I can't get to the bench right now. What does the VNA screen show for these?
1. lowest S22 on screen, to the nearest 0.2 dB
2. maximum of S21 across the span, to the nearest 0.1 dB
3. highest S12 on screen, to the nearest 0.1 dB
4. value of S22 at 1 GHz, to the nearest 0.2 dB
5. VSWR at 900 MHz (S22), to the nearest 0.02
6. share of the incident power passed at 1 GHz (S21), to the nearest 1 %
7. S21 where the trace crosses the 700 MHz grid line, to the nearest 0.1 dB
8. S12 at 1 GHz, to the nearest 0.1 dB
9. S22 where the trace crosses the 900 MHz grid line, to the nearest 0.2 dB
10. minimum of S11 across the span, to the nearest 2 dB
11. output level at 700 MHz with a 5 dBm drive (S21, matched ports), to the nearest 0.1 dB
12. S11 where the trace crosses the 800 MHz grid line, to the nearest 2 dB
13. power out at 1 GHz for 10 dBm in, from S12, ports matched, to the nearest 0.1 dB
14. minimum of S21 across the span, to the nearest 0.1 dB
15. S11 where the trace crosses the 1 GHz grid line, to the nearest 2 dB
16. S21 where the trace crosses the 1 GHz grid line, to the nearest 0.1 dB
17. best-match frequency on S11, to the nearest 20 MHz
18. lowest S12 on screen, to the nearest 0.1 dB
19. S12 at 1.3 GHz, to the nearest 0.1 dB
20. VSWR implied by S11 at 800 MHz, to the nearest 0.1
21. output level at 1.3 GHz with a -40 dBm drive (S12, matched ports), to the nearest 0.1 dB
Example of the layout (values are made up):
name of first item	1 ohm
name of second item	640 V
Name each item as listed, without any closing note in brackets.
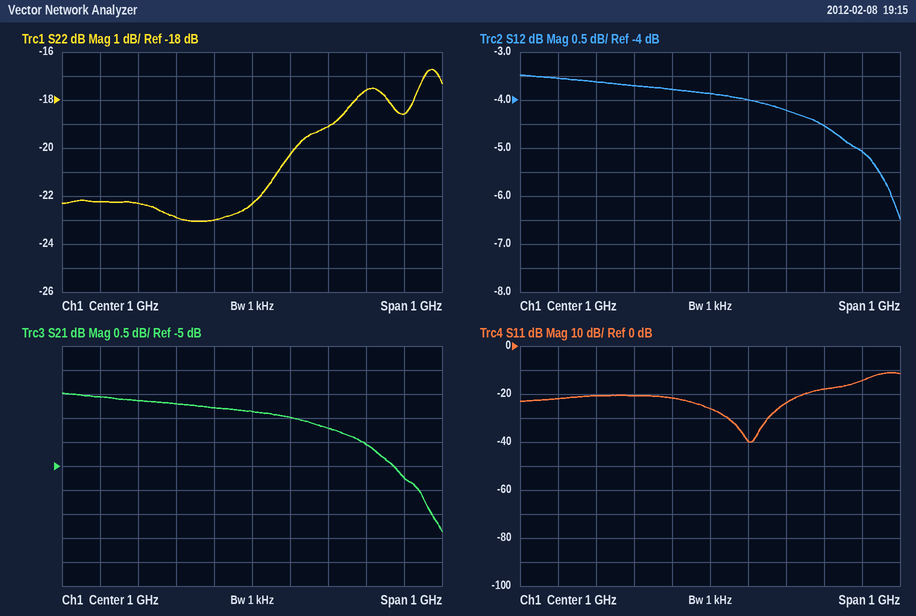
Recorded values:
lowest S22 on screen, to the nearest 0.2 dB	-23.0 dB
maximum of S21 across the span, to the nearest 0.1 dB	-3.5 dB
highest S12 on screen, to the nearest 0.1 dB	-3.5 dB
value of S22 at 1 GHz, to the nearest 0.2 dB	-22.4 dB
VSWR at 900 MHz (S22), to the nearest 0.02	1.16
share of the incident power passed at 1 GHz (S21), to the nearest 1 %	41 %
S21 where the trace crosses the 700 MHz grid line, to the nearest 0.1 dB	-3.6 dB
S12 at 1 GHz, to the nearest 0.1 dB	-3.9 dB
S22 where the trace crosses the 900 MHz grid line, to the nearest 0.2 dB	-23.0 dB
minimum of S11 across the span, to the nearest 2 dB	-40 dB
output level at 700 MHz with a 5 dBm drive (S21, matched ports), to the nearest 0.1 dB	1.4 dBm
S11 where the trace crosses the 800 MHz grid line, to the nearest 2 dB	-20 dB
power out at 1 GHz for 10 dBm in, from S12, ports matched, to the nearest 0.1 dB	6.1 dBm
minimum of S21 across the span, to the nearest 0.1 dB	-6.4 dB
S11 where the trace crosses the 1 GHz grid line, to the nearest 2 dB	-26 dB
S21 where the trace crosses the 1 GHz grid line, to the nearest 0.1 dB	-3.9 dB
best-match frequency on S11, to the nearest 20 MHz	1.10 GHz
lowest S12 on screen, to the nearest 0.1 dB	-6.5 dB
S12 at 1.3 GHz, to the nearest 0.1 dB	-4.5 dB
VSWR implied by S11 at 800 MHz, to the nearest 0.1	1.2
output level at 1.3 GHz with a -40 dBm drive (S12, matched ports), to the nearest 0.1 dB	-44.5 dBm
